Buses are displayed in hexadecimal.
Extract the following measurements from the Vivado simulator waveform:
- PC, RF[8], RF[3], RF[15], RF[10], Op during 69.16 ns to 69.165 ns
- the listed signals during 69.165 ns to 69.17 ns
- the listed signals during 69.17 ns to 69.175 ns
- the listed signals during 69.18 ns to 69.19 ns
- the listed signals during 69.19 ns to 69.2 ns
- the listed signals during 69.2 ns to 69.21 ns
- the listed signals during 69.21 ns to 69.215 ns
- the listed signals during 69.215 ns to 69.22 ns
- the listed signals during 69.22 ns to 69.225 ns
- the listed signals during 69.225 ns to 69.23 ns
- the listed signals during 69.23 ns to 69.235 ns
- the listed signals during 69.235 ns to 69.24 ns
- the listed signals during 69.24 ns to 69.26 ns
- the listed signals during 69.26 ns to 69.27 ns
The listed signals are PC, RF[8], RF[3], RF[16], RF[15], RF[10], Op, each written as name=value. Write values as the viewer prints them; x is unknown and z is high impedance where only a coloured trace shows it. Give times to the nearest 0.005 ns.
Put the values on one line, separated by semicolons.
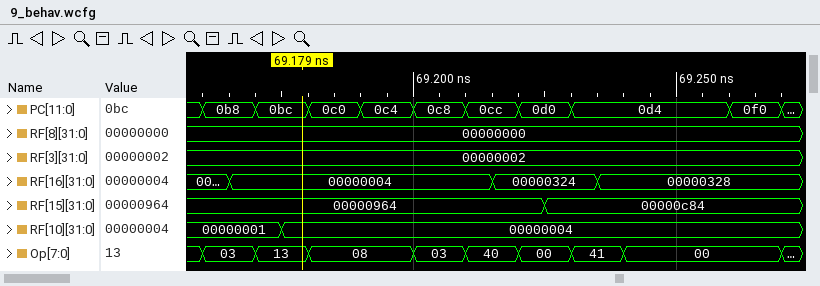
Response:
PC=0b8, RF[8]=00000000, RF[3]=00000002, RF[15]=00000964, RF[10]=00000001, Op=03; PC=0b8, RF[8]=00000000, RF[3]=00000002, RF[16]=00000004, RF[15]=00000964, RF[10]=00000001, Op=03; PC=0bc, RF[8]=00000000, RF[3]=00000002, RF[16]=00000004, RF[15]=00000964, RF[10]=00000001, Op=13; PC=0c0, RF[8]=00000000, RF[3]=00000002, RF[16]=00000004, RF[15]=00000964, RF[10]=00000004, Op=08; PC=0c4, RF[8]=00000000, RF[3]=00000002, RF[16]=00000004, RF[15]=00000964, RF[10]=00000004, Op=08; PC=0c8, RF[8]=00000000, RF[3]=00000002, RF[16]=00000004, RF[15]=00000964, RF[10]=00000004, Op=03; PC=0cc, RF[8]=00000000, RF[3]=00000002, RF[16]=00000004, RF[15]=00000964, RF[10]=00000004, Op=40; PC=0cc, RF[8]=00000000, RF[3]=00000002, RF[16]=00000324, RF[15]=00000964, RF[10]=00000004, Op=40; PC=0d0, RF[8]=00000000, RF[3]=00000002, RF[16]=00000324, RF[15]=00000964, RF[10]=00000004, Op=00; PC=0d0, RF[8]=00000000, RF[3]=00000002, RF[16]=00000324, RF[15]=00000c84, RF[10]=00000004, Op=00; PC=0d4, RF[8]=00000000, RF[3]=00000002, RF[16]=00000324, RF[15]=00000c84, RF[10]=00000004, Op=41; PC=0d4, RF[8]=00000000, RF[3]=00000002, RF[16]=00000328, RF[15]=00000c84, RF[10]=00000004, Op=41; PC=0d4, RF[8]=00000000, RF[3]=00000002, RF[16]=00000328, RF[15]=00000c84, RF[10]=00000004, Op=00; PC=0f0, RF[8]=00000000, RF[3]=00000002, RF[16]=00000328, RF[15]=00000c84, RF[10]=00000004, Op=00
